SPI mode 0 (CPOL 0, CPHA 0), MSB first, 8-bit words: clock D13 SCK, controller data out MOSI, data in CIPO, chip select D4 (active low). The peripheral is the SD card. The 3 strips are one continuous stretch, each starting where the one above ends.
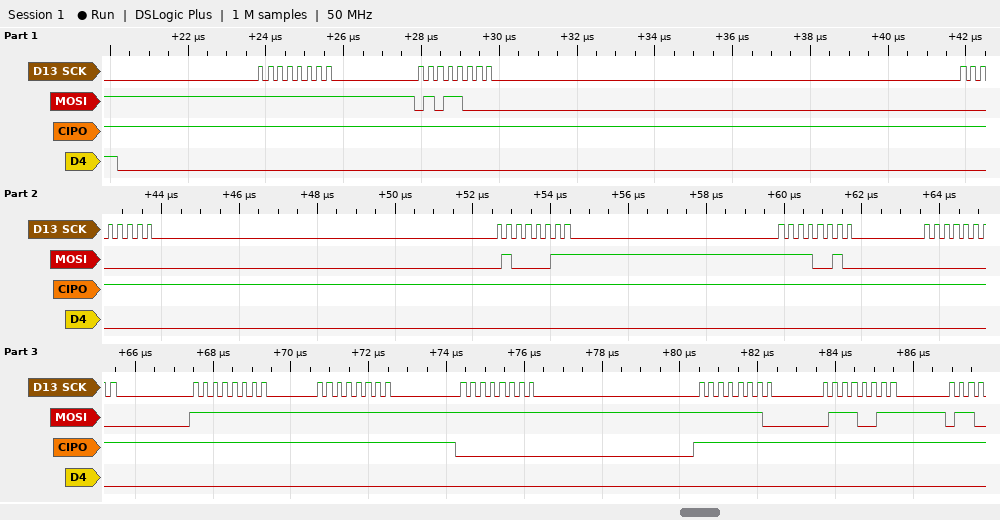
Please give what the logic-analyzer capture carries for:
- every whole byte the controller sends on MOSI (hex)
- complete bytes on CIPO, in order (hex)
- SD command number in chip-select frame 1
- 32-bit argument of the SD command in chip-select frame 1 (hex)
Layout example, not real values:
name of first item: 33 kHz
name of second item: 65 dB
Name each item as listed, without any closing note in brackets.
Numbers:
every whole byte the controller sends on MOSI: FF 58 00 43 F2 00 FF FF FF FE 73
complete bytes on CIPO, in order: FF FF FF FF FF FF FF FF 00 FF FF
SD command number in chip-select frame 1: CMD24
32-bit argument of the SD command in chip-select frame 1: 0x0043F200
